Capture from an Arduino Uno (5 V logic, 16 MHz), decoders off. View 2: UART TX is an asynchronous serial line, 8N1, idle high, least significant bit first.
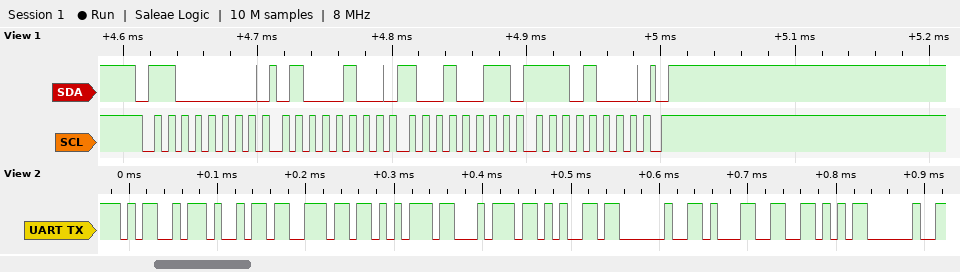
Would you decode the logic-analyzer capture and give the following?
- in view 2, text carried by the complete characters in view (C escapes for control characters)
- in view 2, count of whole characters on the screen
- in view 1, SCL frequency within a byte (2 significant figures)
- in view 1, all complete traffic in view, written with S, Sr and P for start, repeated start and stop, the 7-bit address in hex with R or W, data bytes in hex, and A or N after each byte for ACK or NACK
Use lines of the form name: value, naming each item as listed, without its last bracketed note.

in view 2, text carried by the complete characters in view: "Minute 1V "
in view 2, count of whole characters on the screen: 10
in view 1, SCL frequency within a byte: 100 kHz
in view 1, all complete traffic in view, written with S, Sr and P for start, repeated start and stop, the 7-bit address in hex with R or W, data bytes in hex, and A or N after each byte for ACK or NACK: S 60W A 44 A 93 A E8 A P
